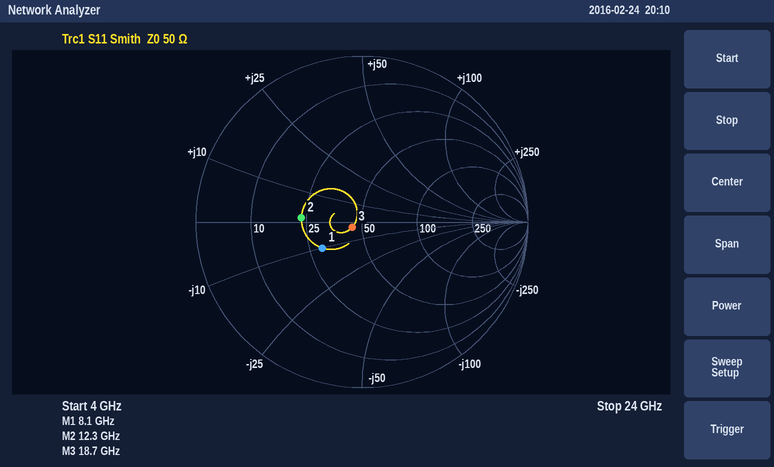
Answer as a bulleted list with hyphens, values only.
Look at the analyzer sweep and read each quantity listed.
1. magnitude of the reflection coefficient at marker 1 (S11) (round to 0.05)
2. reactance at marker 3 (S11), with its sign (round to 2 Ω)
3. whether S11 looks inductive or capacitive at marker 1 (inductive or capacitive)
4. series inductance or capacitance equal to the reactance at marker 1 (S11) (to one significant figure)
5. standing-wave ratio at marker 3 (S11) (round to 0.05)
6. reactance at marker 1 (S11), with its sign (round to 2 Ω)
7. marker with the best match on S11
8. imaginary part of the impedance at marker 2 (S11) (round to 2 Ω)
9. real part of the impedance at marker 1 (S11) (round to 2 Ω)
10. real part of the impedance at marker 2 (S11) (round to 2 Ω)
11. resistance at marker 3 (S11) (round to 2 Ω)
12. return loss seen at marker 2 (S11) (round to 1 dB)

- 0.30
- -2 Ω
- capacitive
- 2 pF
- 1.15
- -10 Ω
- marker 3
- +2 Ω
- 30 Ω
- 24 Ω
- 44 Ω
- 9 dB
